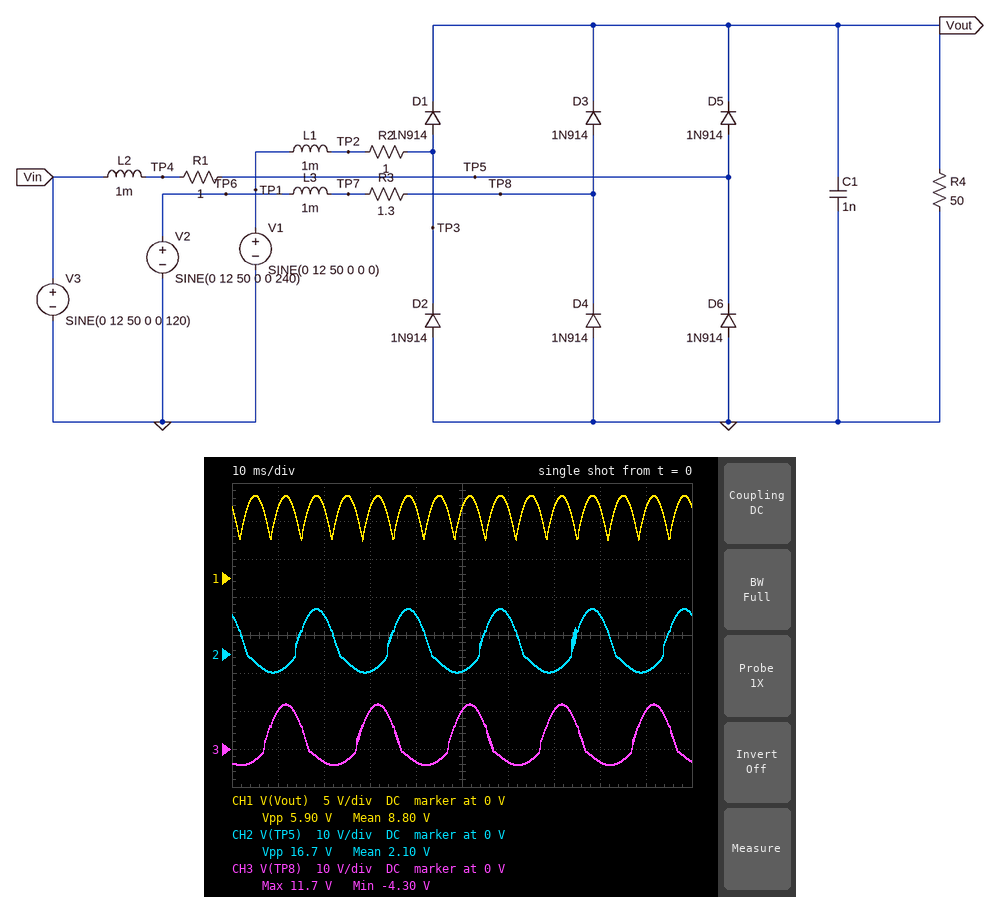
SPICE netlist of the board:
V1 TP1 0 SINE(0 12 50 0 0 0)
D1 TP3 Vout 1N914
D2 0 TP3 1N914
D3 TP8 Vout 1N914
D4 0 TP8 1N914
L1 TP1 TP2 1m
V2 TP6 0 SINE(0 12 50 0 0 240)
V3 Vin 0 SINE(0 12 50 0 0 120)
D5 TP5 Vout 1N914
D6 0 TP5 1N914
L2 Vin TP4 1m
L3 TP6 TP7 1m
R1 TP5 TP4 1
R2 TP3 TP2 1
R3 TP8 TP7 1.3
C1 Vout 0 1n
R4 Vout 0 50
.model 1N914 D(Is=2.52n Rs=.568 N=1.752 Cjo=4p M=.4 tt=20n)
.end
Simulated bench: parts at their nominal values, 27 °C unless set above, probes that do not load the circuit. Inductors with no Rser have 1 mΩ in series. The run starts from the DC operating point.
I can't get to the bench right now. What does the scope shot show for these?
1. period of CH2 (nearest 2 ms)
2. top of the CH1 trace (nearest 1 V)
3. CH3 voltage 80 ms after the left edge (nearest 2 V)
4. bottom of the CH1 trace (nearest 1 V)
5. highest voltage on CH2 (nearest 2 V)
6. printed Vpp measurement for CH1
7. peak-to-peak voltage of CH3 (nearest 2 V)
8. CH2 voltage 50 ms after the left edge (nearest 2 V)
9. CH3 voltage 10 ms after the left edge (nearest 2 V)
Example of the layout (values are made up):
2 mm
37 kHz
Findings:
20 ms
11 V
-4 V
5 V
12 V
5.90 V
16 V
-4 V
10 V
